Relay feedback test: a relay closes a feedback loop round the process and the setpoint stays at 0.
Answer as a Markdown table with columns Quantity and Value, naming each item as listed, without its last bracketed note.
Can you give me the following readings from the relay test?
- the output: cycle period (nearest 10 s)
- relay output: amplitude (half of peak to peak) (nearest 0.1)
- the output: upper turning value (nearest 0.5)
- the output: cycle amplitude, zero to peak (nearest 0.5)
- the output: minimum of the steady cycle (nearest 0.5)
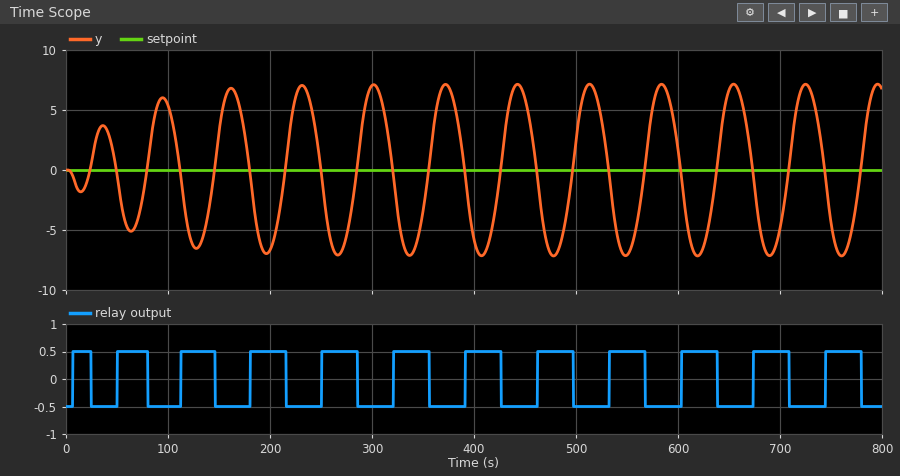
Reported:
| Quantity | Value |
|---|---|
| the output: cycle period | 70 s |
| relay output: amplitude (half of peak to peak) | 0.5 |
| the output: upper turning value | 7.0 |
| the output: cycle amplitude, zero to peak | 7.0 |
| the output: minimum of the steady cycle | -7.0 |
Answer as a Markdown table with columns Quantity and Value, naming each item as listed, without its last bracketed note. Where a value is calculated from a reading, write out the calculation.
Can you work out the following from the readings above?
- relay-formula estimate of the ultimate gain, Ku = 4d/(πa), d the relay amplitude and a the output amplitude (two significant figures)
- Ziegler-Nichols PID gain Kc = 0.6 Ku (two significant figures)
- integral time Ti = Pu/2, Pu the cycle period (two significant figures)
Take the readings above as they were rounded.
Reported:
| Quantity | Value |
|---|---|
| relay-formula estimate of the ultimate gain, Ku = 4d/(πa), d the relay amplitude and a the output amplitude | 4 × 0.5 / (π × 7) = 0.091 |
| Ziegler-Nichols PID gain Kc = 0.6 Ku | 0.6 × 0.091 = 0.055 |
| integral time Ti = Pu/2, Pu the cycle period | 70 / 2 = 35 s |
